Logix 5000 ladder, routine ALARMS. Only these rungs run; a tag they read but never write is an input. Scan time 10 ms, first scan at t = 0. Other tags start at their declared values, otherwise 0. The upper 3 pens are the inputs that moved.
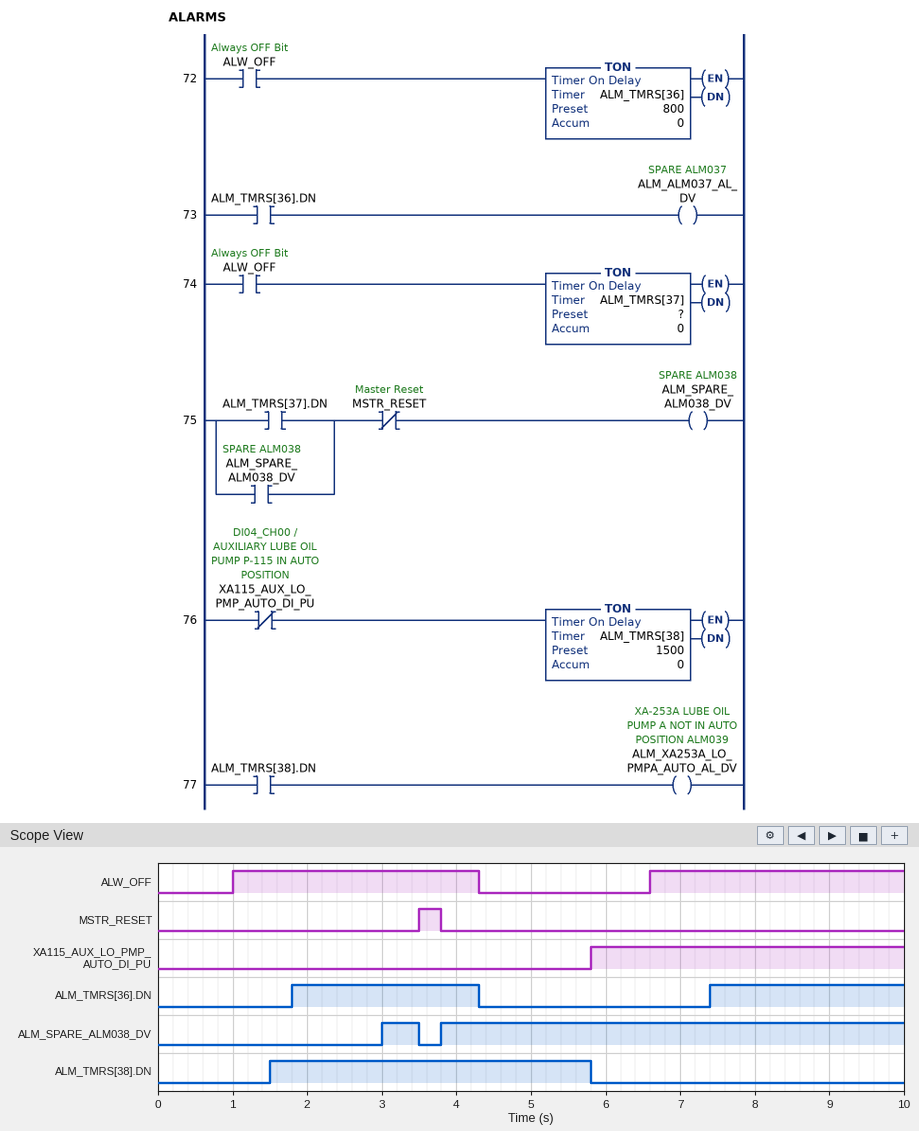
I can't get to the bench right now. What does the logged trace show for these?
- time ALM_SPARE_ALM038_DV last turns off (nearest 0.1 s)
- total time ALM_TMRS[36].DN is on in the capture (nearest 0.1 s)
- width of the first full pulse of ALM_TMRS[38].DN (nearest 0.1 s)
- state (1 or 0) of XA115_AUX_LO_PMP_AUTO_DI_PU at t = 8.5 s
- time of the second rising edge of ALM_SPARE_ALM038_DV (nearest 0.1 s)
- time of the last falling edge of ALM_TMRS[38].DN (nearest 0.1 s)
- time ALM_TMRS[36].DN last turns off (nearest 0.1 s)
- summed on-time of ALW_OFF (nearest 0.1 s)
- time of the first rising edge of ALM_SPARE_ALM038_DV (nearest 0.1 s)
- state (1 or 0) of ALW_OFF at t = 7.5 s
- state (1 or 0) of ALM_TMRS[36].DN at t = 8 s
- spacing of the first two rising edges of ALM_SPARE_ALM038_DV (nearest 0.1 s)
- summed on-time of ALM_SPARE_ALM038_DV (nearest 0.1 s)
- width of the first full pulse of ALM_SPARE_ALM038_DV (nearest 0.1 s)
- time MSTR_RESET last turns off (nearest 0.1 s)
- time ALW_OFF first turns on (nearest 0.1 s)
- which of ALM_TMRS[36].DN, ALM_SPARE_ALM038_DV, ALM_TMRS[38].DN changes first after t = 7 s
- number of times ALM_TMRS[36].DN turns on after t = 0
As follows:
3.5 s
5.1 s
4.3 s
1
3.8 s
5.8 s
4.3 s
6.7 s
3.0 s
1
1
0.8 s
6.7 s
0.5 s
3.8 s
1.0 s
ALM_TMRS[36].DN
2
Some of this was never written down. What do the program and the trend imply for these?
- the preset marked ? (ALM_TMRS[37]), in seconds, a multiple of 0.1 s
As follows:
2.0 s
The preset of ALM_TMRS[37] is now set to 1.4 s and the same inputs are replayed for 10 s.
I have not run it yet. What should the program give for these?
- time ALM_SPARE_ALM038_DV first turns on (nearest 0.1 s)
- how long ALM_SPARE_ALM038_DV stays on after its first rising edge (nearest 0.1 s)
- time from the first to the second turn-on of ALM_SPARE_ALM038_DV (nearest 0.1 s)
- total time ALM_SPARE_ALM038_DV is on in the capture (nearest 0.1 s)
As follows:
2.4 s
1.1 s
1.4 s
7.3 s
